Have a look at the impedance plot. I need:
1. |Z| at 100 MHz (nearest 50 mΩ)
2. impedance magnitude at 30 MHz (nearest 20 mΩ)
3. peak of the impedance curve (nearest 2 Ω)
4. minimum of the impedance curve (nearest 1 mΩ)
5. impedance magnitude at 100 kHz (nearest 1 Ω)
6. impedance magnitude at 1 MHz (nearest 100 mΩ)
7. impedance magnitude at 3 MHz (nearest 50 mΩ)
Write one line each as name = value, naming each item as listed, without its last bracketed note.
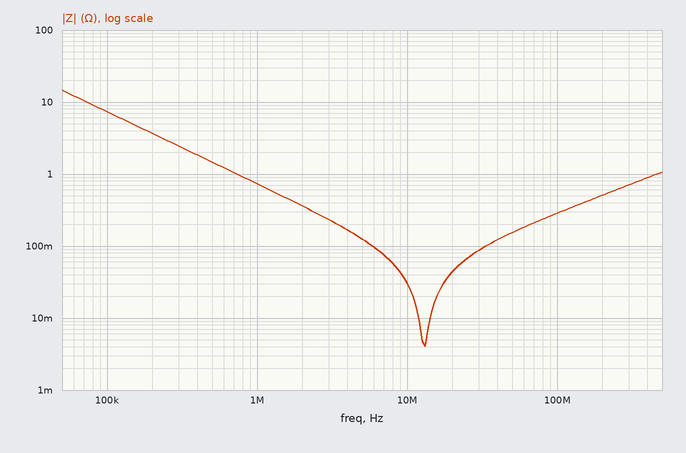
|Z| at 100 MHz = 300 mΩ
impedance magnitude at 30 MHz = 80 mΩ
peak of the impedance curve = 14 Ω
minimum of the impedance curve = 4 mΩ
impedance magnitude at 100 kHz = 7 Ω
impedance magnitude at 1 MHz = 700 mΩ
impedance magnitude at 3 MHz = 250 mΩ
